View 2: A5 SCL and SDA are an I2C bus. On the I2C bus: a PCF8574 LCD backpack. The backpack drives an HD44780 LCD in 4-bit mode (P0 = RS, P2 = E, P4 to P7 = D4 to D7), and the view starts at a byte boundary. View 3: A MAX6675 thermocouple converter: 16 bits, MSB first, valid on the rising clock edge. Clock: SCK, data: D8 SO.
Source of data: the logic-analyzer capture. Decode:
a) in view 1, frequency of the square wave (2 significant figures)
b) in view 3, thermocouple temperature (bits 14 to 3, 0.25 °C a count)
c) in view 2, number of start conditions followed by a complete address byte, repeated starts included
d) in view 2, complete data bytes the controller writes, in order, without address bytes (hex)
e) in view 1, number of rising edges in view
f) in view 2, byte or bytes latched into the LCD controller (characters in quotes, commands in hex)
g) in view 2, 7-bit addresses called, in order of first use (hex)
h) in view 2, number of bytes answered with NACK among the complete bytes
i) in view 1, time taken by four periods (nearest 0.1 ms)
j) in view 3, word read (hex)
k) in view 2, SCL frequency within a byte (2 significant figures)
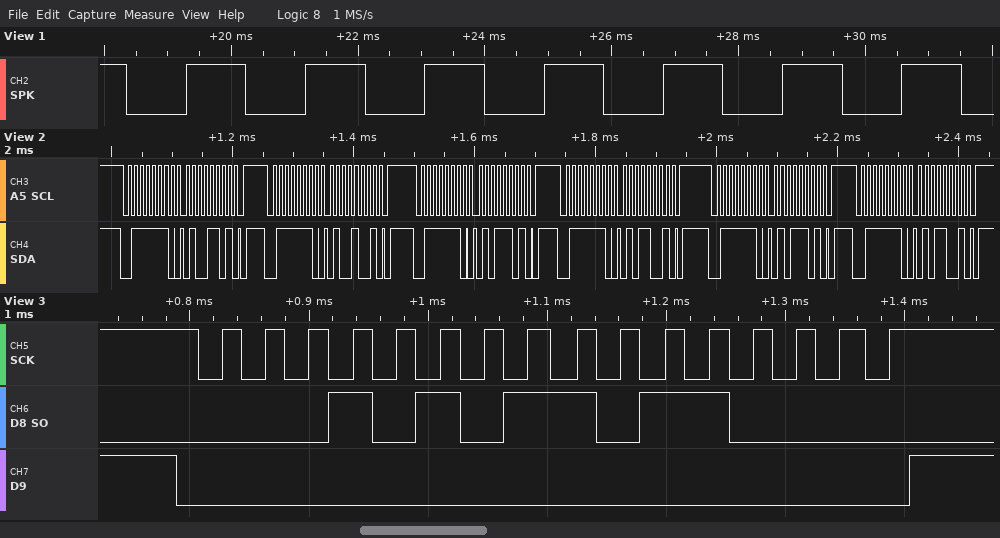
530 Hz
173.50 °C
6
4D 49 5D 59 5D 59
7
'E'
0x3F
0
7.5 ms
0x15B0
100 kHz
